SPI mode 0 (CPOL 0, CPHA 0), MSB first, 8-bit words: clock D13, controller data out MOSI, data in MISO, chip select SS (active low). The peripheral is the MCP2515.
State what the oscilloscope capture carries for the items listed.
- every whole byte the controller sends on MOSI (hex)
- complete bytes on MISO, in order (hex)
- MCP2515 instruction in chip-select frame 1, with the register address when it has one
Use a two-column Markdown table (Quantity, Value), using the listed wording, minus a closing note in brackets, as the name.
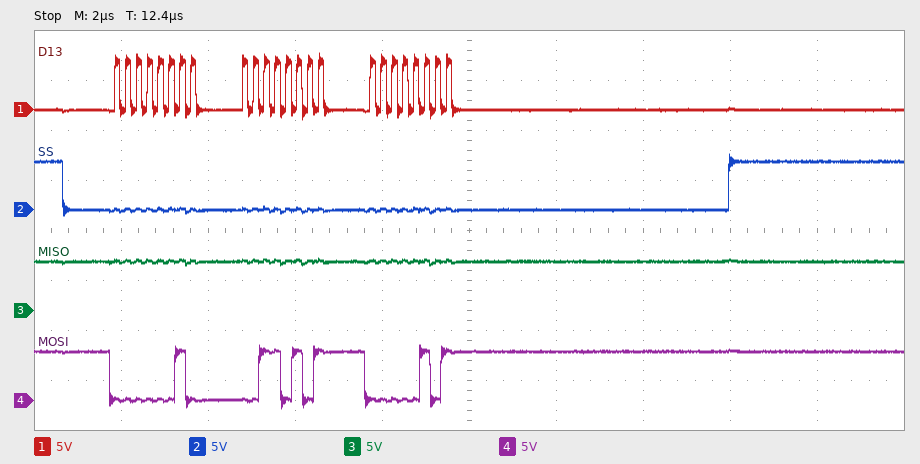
| Quantity | Value |
|---|---|
| every whole byte the controller sends on MOSI | 02 35 05 |
| complete bytes on MISO, in order | FF FF FF |
| MCP2515 instruction in chip-select frame 1, with the register address when it has one | WRITE 0x35 |
